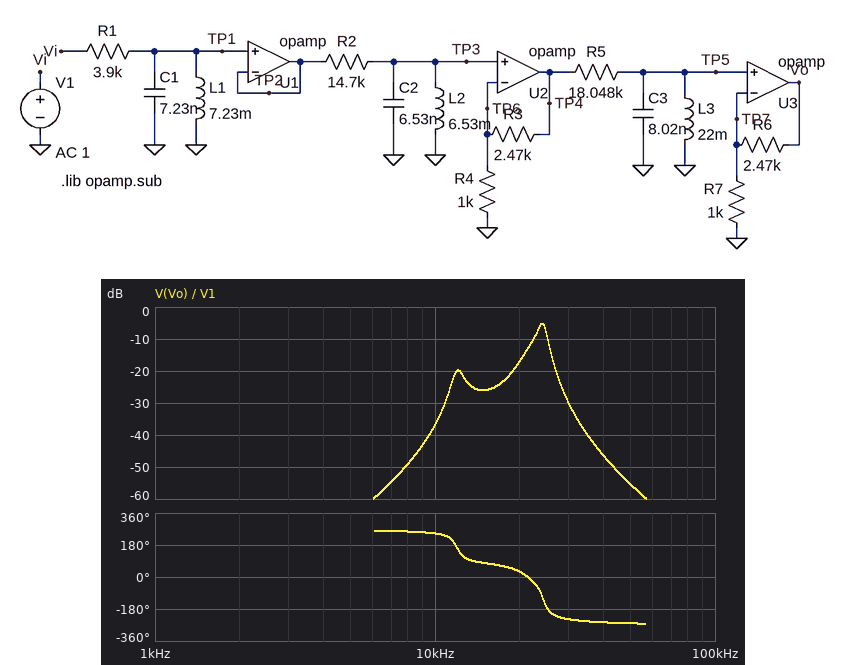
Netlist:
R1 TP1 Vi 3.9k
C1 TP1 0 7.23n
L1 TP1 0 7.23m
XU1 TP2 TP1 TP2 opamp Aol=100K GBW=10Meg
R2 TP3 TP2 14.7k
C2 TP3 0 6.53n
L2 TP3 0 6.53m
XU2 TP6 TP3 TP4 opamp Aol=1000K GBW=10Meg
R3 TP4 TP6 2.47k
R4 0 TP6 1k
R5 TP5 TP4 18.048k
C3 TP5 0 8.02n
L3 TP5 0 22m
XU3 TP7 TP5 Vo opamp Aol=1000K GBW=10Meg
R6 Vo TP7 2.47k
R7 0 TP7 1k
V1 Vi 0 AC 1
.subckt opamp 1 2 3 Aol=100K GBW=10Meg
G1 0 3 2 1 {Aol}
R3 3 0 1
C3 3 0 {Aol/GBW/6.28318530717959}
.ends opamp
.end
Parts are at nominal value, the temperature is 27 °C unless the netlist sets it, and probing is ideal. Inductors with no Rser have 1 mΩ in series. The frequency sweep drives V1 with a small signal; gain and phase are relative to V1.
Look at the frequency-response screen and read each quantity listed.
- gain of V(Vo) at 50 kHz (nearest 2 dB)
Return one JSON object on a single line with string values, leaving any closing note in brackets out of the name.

{"gain of V(Vo) at 50 kHz": "-56 dB"}
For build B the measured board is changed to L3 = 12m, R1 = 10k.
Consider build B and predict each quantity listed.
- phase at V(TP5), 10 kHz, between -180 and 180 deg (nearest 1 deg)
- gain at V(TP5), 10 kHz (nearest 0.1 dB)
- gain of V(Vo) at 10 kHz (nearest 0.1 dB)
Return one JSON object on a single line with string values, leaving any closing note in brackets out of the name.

{"phase at V(TP5), 10 kHz, between -180 and 180 deg": "-99 deg", "gain at V(TP5), 10 kHz": "-67.0 dB", "gain of V(Vo) at 10 kHz": "-56.2 dB"}
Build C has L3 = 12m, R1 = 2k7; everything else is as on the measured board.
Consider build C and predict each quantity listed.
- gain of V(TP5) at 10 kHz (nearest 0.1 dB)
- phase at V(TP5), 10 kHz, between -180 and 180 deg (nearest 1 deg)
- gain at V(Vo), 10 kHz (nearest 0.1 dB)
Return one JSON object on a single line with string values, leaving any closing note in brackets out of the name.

{"gain of V(TP5) at 10 kHz": "-55.8 dB", "phase at V(TP5), 10 kHz, between -180 and 180 deg": "-108 deg", "gain at V(Vo), 10 kHz": "-45.0 dB"}
